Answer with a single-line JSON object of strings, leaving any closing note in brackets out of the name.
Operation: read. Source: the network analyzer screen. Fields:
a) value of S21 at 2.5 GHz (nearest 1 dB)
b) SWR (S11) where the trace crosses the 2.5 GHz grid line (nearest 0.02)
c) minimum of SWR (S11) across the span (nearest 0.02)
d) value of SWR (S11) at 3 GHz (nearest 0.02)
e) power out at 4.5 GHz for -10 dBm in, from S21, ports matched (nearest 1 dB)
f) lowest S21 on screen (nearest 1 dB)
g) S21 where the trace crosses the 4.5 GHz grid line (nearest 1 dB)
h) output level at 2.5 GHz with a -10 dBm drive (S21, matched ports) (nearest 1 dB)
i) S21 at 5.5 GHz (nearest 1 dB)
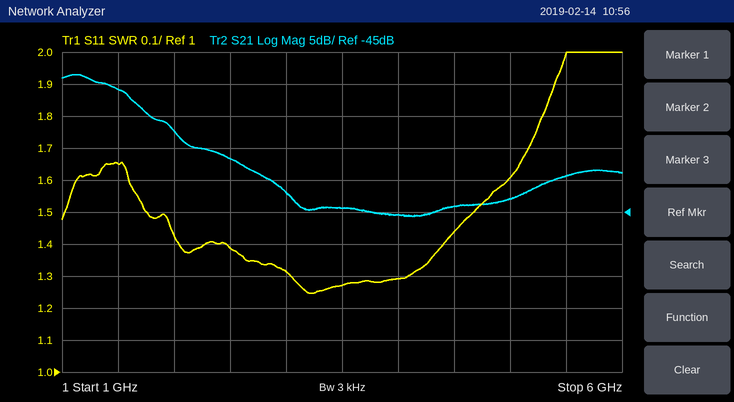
{"value of S21 at 2.5 GHz": "-37 dB", "SWR (S11) where the trace crosses the 2.5 GHz grid line": "1.38", "minimum of SWR (S11) across the span": "1.24", "value of SWR (S11) at 3 GHz": "1.32", "power out at 4.5 GHz for -10 dBm in, from S21, ports matched": "-54 dBm", "lowest S21 on screen": "-46 dB", "S21 where the trace crosses the 4.5 GHz grid line": "-44 dB", "output level at 2.5 GHz with a -10 dBm drive (S21, matched ports)": "-47 dBm", "S21 at 5.5 GHz": "-39 dB"}
